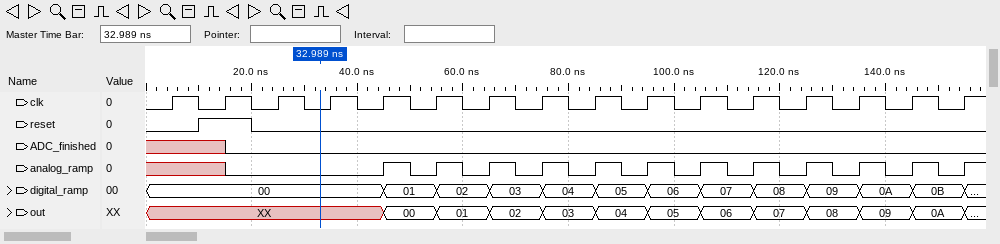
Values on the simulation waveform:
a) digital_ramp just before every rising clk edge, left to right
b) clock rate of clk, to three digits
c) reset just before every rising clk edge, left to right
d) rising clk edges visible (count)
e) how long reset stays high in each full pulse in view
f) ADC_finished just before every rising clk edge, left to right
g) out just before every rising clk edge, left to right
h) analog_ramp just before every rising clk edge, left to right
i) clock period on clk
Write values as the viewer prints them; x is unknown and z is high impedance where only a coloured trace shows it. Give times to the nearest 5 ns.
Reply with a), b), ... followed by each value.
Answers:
a) 00, 00, 00, 00, 00, 01, 02, 03, 04, 05, 06, 07, 08, 09, 0A, 0B
b) 100 MHz
c) 0 1 0 0 0 0 0 0 0 0 0 0 0 0 0 0
d) 16
e) 10 ns
f) x x 0 0 0 0 0 0 0 0 0 0 0 0 0 0
g) XX, XX, XX, XX, XX, 00, 01, 02, 03, 04, 05, 06, 07, 08, 09, 0A
h) x x 0 0 0 0 0 0 0 0 0 0 0 0 0 0
i) 10 ns
